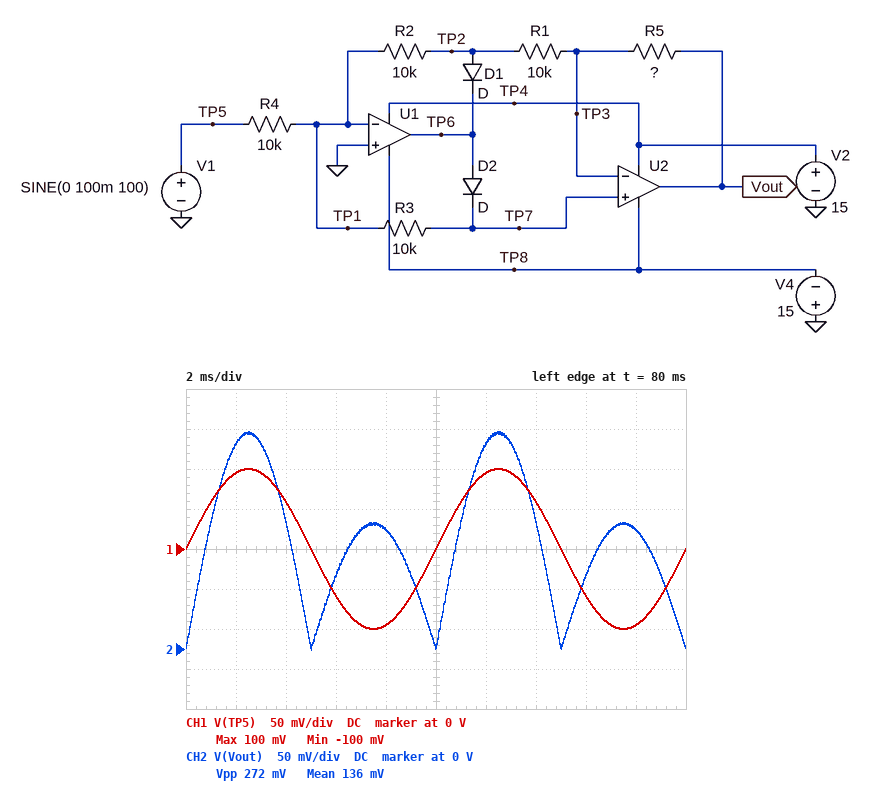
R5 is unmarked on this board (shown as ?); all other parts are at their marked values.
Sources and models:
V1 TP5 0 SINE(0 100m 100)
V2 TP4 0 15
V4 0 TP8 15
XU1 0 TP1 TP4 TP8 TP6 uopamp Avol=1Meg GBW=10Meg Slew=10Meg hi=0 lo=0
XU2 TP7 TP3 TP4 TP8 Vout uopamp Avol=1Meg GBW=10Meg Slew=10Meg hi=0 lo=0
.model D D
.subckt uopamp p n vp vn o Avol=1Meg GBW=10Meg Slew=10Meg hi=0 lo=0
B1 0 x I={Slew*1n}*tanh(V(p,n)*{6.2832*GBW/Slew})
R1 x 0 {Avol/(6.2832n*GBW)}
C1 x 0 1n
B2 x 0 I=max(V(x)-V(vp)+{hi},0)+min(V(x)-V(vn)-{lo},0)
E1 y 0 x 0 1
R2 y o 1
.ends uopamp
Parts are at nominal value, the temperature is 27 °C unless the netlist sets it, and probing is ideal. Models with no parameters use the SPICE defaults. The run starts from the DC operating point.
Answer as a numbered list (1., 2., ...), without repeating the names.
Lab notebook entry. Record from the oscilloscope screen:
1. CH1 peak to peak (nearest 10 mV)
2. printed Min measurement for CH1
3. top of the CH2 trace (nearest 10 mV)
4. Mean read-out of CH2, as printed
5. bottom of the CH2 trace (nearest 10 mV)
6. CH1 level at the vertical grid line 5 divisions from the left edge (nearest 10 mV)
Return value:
1. 200 mV
2. -100 mV
3. 270 mV
4. 136 mV
5. 0 V
6. 0 V
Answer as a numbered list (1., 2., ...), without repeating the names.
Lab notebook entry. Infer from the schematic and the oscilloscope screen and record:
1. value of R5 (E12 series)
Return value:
1. 27 kΩ
